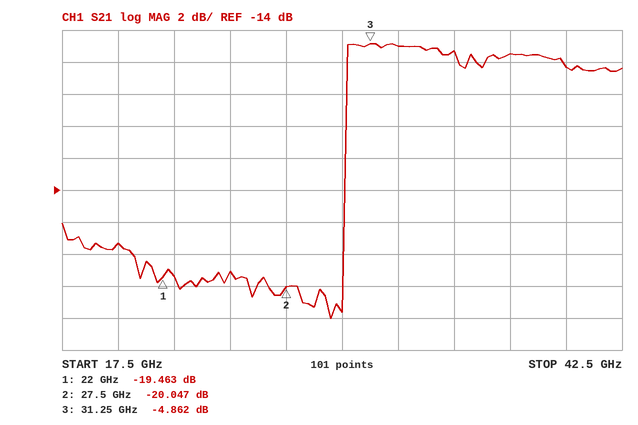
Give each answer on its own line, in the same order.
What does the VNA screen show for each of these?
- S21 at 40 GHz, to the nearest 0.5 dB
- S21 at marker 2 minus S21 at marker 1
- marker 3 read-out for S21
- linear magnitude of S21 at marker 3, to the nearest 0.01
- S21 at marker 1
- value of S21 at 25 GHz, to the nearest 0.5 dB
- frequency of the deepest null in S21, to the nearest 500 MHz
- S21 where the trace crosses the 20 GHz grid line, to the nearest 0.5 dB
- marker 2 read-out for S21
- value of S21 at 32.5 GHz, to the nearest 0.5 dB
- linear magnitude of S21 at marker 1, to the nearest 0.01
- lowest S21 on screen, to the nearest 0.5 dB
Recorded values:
-6.5 dB
-0.584 dB
-4.862 dB
0.57
-19.463 dB
-19.0 dB
29.5 GHz
-17.5 dB
-20.047 dB
-5.0 dB
0.11
-22.0 dB
